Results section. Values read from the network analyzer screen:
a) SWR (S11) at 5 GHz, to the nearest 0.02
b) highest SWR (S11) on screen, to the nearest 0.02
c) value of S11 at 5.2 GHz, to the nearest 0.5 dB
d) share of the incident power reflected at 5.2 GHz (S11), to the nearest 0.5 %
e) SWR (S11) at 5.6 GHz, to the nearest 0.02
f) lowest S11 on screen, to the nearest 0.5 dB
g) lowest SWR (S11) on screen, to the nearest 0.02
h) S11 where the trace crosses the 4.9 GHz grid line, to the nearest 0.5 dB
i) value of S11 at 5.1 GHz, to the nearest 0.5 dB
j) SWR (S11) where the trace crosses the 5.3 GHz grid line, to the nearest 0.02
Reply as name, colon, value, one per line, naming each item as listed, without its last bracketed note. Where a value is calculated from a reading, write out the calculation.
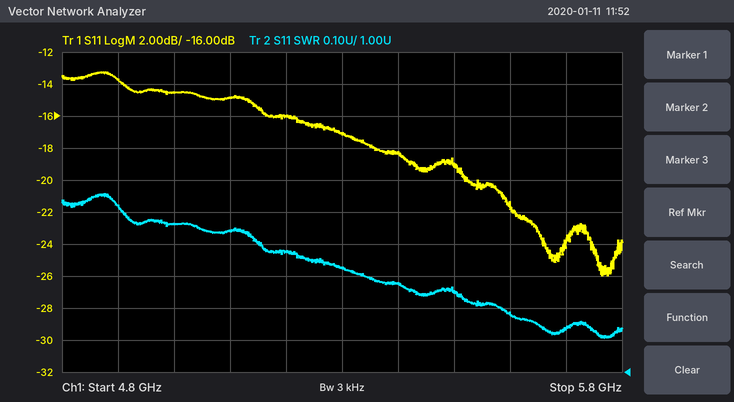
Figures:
SWR (S11) at 5 GHz, to the nearest 0.02: 1.46
highest SWR (S11) on screen, to the nearest 0.02: 1.56
value of S11 at 5.2 GHz, to the nearest 0.5 dB: -16.0 dB
share of the incident power reflected at 5.2 GHz (S11), to the nearest 0.5 %: 10^(-16/10) ≈ 2.5 %
SWR (S11) at 5.6 GHz, to the nearest 0.02: 1.18
lowest S11 on screen, to the nearest 0.5 dB: -26.0 dB
lowest SWR (S11) on screen, to the nearest 0.02: 1.10
S11 where the trace crosses the 4.9 GHz grid line, to the nearest 0.5 dB: -13.5 dB
value of S11 at 5.1 GHz, to the nearest 0.5 dB: -15.0 dB
SWR (S11) where the trace crosses the 5.3 GHz grid line, to the nearest 0.02: 1.32
